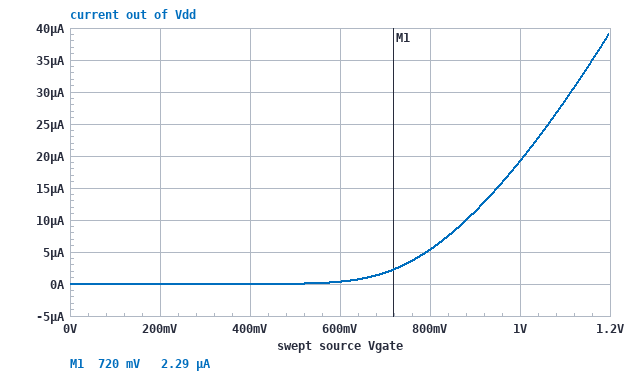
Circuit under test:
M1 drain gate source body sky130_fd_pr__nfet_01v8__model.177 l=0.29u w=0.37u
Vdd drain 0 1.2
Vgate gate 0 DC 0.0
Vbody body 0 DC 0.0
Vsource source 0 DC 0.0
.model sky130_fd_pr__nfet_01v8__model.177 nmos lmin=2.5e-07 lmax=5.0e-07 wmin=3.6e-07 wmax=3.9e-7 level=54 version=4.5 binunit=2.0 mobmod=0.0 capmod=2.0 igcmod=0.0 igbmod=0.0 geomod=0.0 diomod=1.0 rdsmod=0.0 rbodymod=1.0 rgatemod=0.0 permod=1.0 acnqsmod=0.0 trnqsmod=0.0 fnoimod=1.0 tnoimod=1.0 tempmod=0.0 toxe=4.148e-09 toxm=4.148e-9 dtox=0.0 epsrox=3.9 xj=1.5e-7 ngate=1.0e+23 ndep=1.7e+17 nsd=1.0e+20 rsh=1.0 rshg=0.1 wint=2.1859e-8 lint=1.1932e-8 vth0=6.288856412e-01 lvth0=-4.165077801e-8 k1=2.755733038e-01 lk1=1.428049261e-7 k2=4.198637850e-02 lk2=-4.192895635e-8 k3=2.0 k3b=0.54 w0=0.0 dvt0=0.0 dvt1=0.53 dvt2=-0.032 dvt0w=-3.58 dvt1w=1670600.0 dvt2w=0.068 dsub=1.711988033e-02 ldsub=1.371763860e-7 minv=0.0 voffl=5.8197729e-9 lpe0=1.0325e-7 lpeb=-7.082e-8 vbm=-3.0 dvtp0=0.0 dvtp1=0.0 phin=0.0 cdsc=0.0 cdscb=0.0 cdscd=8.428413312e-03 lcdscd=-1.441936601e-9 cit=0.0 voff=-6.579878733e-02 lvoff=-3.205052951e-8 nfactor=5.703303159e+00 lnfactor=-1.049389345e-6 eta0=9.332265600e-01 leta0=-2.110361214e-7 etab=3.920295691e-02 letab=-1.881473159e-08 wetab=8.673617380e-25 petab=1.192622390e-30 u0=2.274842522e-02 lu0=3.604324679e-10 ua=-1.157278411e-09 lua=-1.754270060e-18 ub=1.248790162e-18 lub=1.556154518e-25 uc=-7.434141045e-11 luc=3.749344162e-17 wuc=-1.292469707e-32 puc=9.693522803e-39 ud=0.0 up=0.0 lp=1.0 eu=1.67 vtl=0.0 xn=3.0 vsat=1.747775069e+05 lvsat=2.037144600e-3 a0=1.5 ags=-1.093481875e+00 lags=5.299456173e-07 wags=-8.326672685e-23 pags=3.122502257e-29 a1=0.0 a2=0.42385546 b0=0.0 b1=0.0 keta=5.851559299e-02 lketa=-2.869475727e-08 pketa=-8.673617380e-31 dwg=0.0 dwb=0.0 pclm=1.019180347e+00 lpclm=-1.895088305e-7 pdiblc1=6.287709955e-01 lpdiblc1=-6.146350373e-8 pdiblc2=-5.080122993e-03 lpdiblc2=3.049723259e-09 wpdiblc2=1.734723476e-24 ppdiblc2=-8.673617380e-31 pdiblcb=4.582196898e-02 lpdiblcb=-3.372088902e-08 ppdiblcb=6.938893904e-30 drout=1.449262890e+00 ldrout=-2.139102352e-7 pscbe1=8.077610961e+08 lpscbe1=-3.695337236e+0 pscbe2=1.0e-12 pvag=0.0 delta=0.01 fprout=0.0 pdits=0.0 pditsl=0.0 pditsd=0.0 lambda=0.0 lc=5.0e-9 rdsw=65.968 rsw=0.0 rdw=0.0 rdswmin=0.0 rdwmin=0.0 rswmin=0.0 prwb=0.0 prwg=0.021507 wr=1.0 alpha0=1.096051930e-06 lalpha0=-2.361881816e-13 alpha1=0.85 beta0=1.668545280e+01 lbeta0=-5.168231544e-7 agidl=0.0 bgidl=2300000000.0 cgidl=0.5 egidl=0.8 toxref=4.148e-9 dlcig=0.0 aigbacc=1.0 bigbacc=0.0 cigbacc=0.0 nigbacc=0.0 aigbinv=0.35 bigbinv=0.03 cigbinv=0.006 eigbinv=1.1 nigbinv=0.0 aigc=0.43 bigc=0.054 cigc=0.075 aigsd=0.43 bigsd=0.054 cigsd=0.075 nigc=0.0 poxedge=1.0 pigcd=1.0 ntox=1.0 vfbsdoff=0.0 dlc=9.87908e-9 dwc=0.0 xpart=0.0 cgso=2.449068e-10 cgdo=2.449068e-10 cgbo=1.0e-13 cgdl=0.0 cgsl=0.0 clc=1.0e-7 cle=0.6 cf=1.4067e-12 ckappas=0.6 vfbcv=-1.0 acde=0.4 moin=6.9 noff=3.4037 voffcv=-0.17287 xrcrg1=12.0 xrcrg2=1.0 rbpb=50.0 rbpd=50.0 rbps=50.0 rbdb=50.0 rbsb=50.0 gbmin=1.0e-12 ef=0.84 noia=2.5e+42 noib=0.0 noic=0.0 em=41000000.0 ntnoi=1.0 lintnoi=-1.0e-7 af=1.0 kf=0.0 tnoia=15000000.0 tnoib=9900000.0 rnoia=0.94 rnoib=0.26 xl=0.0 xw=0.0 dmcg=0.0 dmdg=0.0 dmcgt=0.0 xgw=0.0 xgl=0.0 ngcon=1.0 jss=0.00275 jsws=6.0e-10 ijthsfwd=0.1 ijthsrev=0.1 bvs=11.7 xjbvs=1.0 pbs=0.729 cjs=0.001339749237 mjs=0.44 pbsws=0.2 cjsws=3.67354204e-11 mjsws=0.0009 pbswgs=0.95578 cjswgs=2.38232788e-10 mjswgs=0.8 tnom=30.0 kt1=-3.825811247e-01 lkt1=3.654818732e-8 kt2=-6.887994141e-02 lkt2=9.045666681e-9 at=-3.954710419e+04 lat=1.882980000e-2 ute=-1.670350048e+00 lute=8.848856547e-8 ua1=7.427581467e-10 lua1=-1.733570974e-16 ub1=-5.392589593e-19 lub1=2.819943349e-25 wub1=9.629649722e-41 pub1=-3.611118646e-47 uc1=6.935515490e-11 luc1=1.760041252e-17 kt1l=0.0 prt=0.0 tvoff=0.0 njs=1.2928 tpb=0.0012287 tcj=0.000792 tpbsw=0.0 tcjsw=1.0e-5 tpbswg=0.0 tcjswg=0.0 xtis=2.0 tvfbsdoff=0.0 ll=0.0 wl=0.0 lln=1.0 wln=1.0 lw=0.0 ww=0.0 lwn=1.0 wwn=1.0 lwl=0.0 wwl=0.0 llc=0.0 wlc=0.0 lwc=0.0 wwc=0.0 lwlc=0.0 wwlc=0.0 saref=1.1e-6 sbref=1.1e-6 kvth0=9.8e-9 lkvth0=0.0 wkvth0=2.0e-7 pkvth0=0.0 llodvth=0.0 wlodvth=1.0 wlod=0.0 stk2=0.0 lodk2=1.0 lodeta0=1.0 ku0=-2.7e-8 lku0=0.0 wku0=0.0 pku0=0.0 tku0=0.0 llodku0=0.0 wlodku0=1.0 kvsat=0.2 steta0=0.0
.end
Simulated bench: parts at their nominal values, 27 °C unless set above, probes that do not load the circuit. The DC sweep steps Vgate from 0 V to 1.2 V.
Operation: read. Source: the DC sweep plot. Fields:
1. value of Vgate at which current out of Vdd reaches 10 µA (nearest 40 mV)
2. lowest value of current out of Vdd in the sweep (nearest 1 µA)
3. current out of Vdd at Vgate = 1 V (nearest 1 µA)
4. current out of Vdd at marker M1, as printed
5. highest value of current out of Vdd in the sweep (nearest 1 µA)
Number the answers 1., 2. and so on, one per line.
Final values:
1. 880 mV
2. 0 A
3. 19 µA
4. 2.29 µA
5. 39 µA
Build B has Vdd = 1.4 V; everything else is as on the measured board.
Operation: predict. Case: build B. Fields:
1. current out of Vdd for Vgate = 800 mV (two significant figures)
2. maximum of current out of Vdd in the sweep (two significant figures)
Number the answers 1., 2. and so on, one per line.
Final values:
1. 5.5 µA
2. 40 µA
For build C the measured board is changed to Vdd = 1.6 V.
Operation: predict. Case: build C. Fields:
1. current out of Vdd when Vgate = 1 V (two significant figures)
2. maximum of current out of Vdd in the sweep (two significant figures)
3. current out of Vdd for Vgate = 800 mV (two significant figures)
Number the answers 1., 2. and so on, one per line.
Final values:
1. 20 µA
2. 40 µA
3. 5.6 µA
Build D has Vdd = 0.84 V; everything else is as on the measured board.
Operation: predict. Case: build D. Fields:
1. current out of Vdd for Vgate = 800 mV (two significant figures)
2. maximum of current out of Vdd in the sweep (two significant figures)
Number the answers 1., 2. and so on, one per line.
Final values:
1. 5.1 µA
2. 38 µA
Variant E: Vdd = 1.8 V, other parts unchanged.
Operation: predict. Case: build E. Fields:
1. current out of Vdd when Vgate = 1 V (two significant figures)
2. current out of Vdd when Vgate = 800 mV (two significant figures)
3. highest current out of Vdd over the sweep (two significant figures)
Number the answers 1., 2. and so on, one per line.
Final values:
1. 20 µA
2. 5.7 µA
3. 41 µA
